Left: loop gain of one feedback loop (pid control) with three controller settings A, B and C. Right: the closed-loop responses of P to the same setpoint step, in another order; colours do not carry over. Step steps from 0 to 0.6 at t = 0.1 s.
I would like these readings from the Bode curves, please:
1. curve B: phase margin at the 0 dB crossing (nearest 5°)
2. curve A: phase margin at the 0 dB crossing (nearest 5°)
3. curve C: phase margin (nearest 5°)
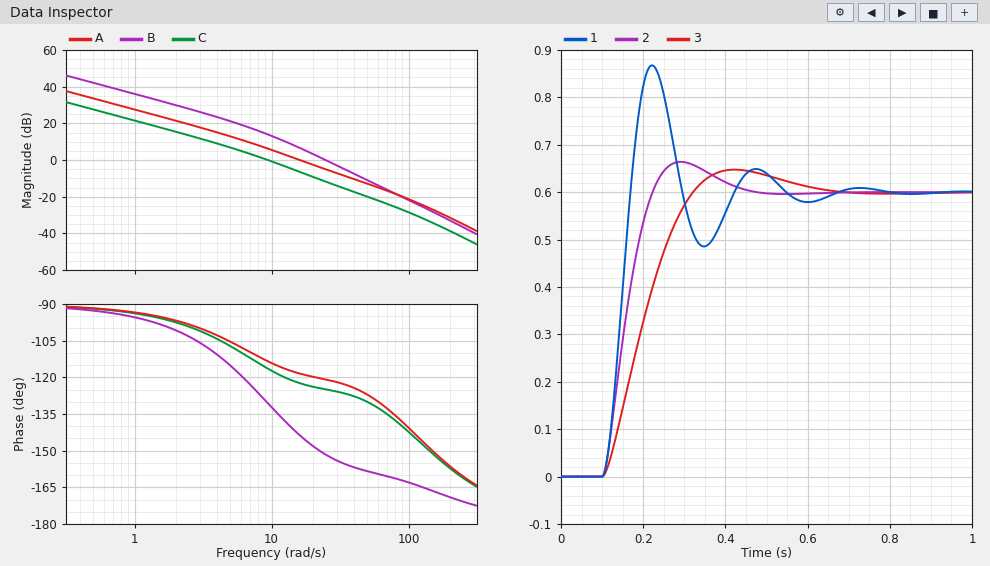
30°
60°
65°
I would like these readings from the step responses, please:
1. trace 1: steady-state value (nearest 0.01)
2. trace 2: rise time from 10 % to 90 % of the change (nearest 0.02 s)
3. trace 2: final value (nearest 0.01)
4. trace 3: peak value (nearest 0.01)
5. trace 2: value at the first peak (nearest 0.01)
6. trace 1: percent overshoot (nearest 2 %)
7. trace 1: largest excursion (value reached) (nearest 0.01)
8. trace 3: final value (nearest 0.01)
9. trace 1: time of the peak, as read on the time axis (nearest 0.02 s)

0.60
0.08 s
0.60
0.65
0.66
44 %
0.87
0.60
0.22 s
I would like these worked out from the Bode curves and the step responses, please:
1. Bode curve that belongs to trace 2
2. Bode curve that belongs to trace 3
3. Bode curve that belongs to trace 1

A
C
B
